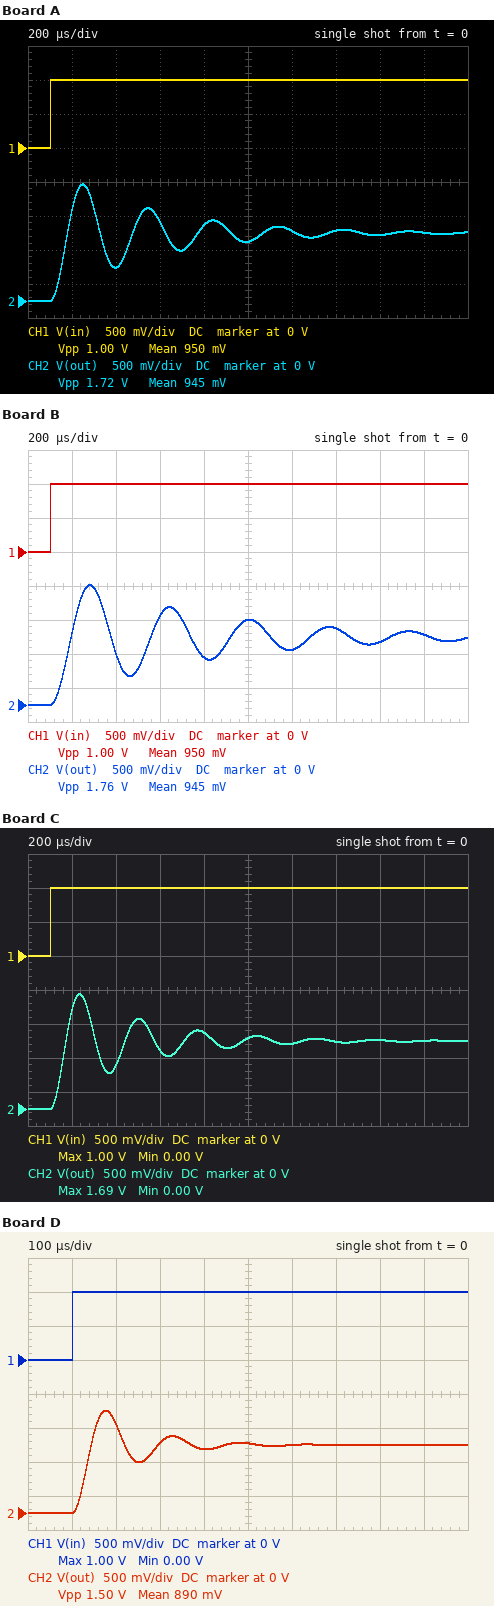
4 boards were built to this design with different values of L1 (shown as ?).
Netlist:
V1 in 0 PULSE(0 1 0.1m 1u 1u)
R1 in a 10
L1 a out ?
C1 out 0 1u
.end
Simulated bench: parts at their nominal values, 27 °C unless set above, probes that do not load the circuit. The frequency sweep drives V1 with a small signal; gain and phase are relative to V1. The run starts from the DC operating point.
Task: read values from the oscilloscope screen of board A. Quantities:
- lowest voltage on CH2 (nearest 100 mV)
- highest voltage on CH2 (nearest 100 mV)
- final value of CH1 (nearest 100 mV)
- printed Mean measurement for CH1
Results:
0 V
1.7 V
1.0 V
950 mV
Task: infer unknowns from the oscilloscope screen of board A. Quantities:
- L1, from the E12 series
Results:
2.2 mH
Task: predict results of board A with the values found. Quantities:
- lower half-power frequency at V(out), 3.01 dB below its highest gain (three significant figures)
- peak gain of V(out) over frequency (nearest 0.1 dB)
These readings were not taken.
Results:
2.97 kHz
13.5 dB
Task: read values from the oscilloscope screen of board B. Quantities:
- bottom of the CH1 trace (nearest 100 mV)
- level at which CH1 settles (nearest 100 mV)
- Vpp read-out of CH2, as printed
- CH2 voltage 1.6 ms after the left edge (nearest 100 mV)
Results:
0 V
1.0 V
1.76 V
900 mV
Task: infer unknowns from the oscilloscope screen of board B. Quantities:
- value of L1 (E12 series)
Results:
3.3 mH
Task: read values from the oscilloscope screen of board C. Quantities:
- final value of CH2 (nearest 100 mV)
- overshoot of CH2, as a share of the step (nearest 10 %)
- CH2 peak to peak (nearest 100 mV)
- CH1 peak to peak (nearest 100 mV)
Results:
1.0 V
70 %
1.7 V
1.0 V
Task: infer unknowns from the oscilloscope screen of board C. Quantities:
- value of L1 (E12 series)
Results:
1.8 mH
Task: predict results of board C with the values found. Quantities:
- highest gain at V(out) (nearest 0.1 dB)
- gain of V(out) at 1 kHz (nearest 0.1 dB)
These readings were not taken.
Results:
12.6 dB
0.6 dB
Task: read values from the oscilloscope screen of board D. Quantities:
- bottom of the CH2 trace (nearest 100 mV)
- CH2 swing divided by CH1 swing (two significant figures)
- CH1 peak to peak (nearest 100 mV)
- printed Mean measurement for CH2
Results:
0 V
1.5
1.0 V
890 mV
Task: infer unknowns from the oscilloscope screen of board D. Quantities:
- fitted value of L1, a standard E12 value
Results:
560 µH
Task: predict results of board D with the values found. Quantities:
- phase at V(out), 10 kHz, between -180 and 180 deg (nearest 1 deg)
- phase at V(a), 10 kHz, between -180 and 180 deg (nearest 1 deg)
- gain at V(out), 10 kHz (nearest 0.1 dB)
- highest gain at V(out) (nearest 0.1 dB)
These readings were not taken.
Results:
-153 deg
27 deg
-2.7 dB
7.7 dB
